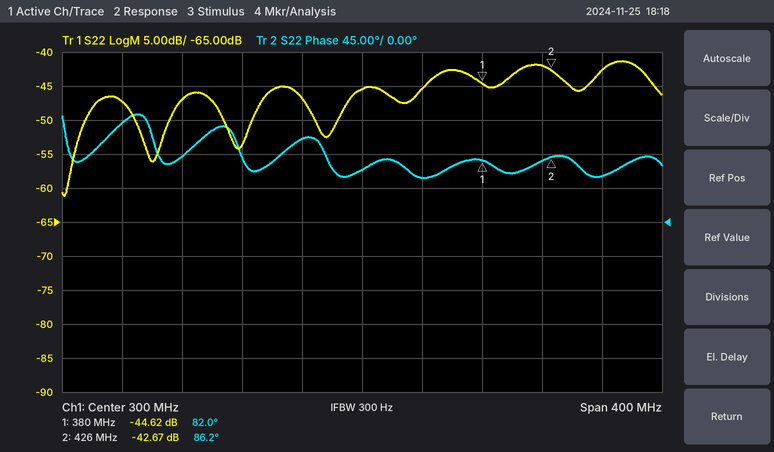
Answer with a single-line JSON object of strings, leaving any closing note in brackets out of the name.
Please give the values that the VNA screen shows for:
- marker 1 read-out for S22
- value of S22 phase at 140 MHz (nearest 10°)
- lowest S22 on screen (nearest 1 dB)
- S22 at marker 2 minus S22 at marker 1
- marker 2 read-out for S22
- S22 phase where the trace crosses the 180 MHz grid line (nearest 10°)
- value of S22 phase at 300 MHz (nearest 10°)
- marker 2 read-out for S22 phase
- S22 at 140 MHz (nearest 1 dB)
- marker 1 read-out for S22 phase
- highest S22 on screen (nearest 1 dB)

{"marker 1 read-out for S22": "-44.62 dB", "value of S22 phase at 140 MHz": "130°", "lowest S22 on screen": "-61 dB", "S22 at marker 2 minus S22 at marker 1": "1.95 dB", "marker 2 read-out for S22": "-42.67 dB", "S22 phase where the trace crosses the 180 MHz grid line": "90°", "value of S22 phase at 300 MHz": "70°", "marker 2 read-out for S22 phase": "86.2°", "S22 at 140 MHz": "-47 dB", "marker 1 read-out for S22 phase": "82.0°", "highest S22 on screen": "-41 dB"}
